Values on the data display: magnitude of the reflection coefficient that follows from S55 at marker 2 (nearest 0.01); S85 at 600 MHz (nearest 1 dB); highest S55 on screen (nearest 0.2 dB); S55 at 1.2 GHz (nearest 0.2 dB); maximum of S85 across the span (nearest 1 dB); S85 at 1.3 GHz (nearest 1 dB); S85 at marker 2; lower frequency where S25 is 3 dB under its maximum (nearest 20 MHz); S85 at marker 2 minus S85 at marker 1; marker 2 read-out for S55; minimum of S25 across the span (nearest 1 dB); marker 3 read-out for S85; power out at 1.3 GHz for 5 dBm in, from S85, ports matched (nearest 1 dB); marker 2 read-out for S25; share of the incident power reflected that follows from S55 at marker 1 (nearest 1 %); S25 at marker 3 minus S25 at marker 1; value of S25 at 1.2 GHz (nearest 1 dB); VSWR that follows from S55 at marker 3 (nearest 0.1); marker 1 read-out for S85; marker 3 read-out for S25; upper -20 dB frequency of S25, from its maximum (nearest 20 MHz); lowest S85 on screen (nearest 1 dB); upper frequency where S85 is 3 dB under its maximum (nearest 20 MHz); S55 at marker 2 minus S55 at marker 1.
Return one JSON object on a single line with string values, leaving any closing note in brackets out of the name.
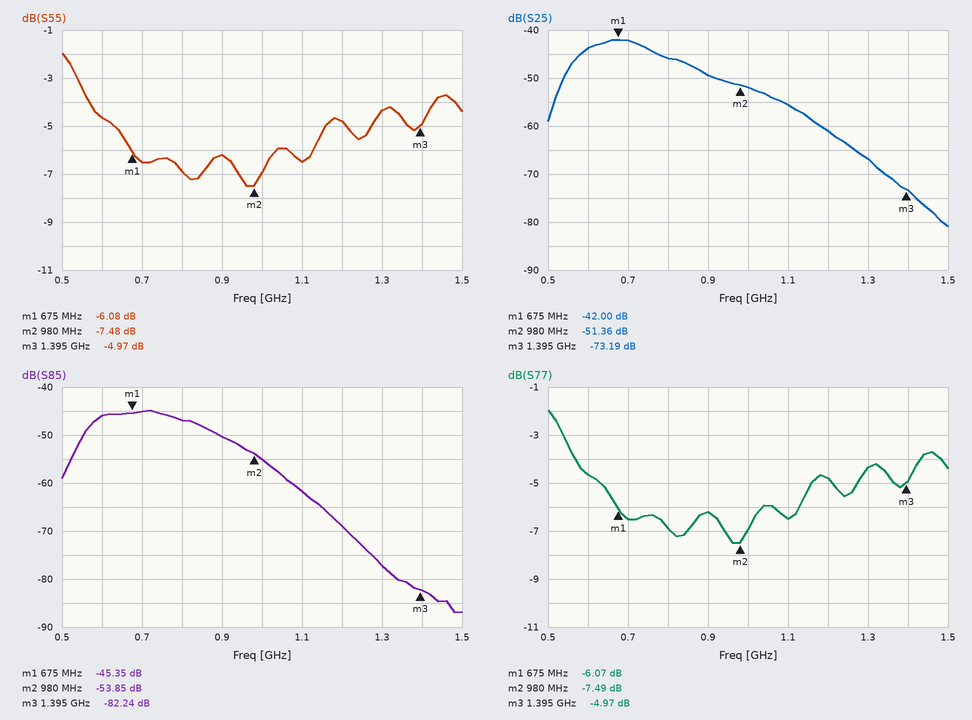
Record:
{"magnitude of the reflection coefficient that follows from S55 at marker 2": "0.42", "S85 at 600 MHz": "-46 dB", "highest S55 on screen": "-2.0 dB", "S55 at 1.2 GHz": "-4.8 dB", "maximum of S85 across the span": "-45 dB", "S85 at 1.3 GHz": "-77 dB", "S85 at marker 2": "-53.85 dB", "lower frequency where S25 is 3 dB under its maximum": "580 MHz", "S85 at marker 2 minus S85 at marker 1": "-8.50 dB", "marker 2 read-out for S55": "-7.48 dB", "minimum of S25 across the span": "-81 dB", "marker 3 read-out for S85": "-82.24 dB", "power out at 1.3 GHz for 5 dBm in, from S85, ports matched": "-72 dBm", "marker 2 read-out for S25": "-51.36 dB", "share of the incident power reflected that follows from S55 at marker 1": "25 %", "S25 at marker 3 minus S25 at marker 1": "-31.19 dB", "value of S25 at 1.2 GHz": "-61 dB", "VSWR that follows from S55 at marker 3": "3.6", "marker 1 read-out for S85": "-45.35 dB", "marker 3 read-out for S25": "-73.19 dB", "upper -20 dB frequency of S25, from its maximum": "1.22 GHz", "lowest S85 on screen": "-87 dB", "upper frequency where S85 is 3 dB under its maximum": "840 MHz", "S55 at marker 2 minus S55 at marker 1": "-1.40 dB"}
